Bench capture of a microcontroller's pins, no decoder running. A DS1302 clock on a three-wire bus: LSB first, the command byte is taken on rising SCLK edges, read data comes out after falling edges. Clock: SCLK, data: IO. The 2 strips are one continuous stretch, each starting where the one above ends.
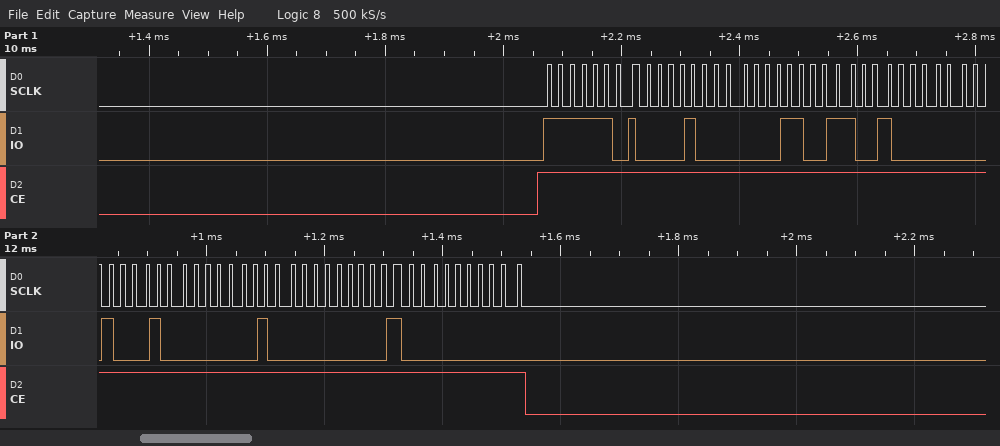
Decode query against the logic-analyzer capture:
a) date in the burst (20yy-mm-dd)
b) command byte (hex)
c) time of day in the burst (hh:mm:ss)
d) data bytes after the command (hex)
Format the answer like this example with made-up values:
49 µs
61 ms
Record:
2020-02-20
0xBF
13:30:10
10 30 13 20 02 04 20 00
